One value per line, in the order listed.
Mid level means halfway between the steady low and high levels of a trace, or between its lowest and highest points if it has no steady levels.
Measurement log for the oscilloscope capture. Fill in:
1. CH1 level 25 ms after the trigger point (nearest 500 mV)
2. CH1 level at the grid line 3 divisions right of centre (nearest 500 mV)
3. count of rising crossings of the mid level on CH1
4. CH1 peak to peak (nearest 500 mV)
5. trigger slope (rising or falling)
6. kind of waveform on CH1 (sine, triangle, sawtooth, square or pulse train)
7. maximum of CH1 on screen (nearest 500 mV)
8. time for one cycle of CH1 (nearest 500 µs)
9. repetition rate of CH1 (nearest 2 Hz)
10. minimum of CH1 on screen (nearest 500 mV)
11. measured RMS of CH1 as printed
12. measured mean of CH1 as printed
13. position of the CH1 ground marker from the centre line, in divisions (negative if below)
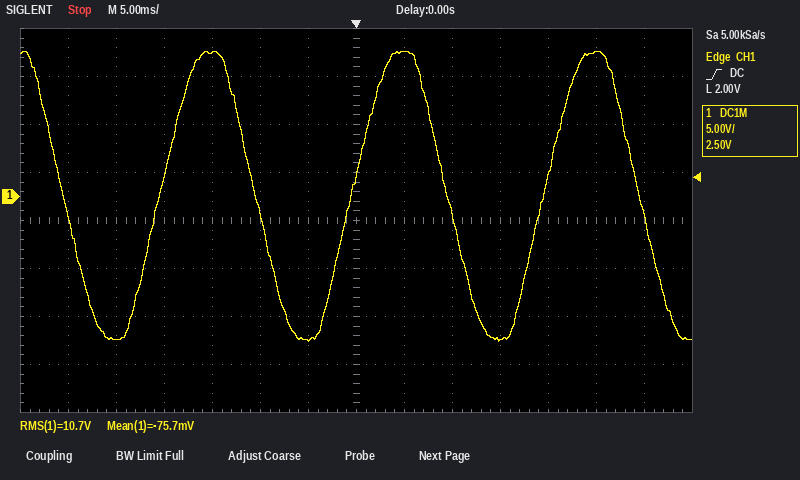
15.0 V
-15.0 V
3
30.0 V
rising
sine
15.0 V
20.0 ms
50 Hz
-15.0 V
10.7 V
-75.7 mV
+0.5 div
